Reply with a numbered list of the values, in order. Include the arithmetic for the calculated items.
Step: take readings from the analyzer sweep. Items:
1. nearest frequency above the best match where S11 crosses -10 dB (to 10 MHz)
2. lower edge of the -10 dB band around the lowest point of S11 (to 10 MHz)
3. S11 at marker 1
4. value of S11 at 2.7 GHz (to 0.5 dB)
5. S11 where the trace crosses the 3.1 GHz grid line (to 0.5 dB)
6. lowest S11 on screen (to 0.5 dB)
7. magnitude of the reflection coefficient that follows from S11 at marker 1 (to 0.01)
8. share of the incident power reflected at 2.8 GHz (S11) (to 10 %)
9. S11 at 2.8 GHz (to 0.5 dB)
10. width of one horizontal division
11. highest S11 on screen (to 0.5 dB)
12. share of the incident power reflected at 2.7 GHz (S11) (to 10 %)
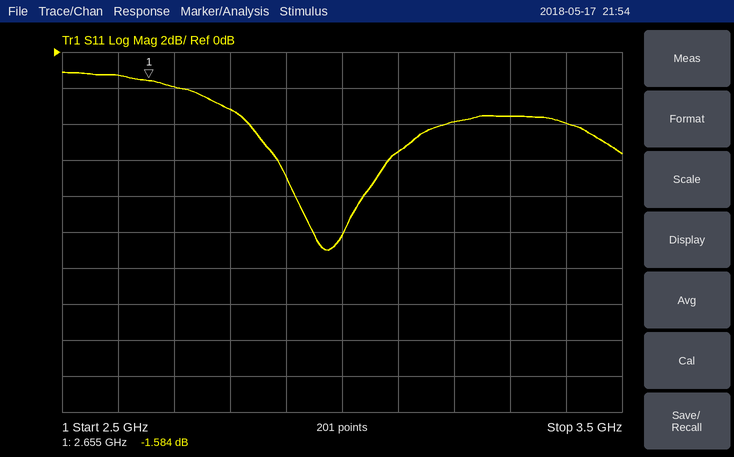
1. 3.00 GHz
2. 2.95 GHz
3. -1.584 dB
4. -2.0 dB
5. -5.5 dB
6. -11.0 dB
7. 10^(-1.584/20) ≈ 0.83
8. 10^(-3/10) ≈ 50 %
9. -3.0 dB
10. 100 MHz
11. -1.0 dB
12. 10^(-2/10) ≈ 63.1 %, so 60 % to the nearest 10 %
